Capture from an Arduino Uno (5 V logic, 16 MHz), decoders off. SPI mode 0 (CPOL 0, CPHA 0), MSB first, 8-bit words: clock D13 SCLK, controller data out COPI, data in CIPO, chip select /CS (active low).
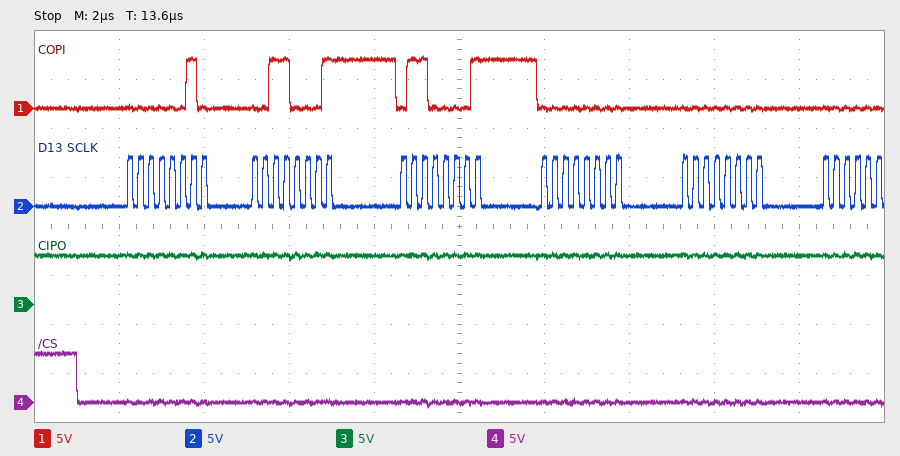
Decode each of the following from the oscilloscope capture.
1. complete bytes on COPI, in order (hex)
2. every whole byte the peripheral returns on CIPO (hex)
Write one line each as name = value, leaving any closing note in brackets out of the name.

complete bytes on COPI, in order = 0x02 0x31 0x61 0x00 0x00
every whole byte the peripheral returns on CIPO = 0xFF 0xFF 0xFF 0xFF 0xFF
